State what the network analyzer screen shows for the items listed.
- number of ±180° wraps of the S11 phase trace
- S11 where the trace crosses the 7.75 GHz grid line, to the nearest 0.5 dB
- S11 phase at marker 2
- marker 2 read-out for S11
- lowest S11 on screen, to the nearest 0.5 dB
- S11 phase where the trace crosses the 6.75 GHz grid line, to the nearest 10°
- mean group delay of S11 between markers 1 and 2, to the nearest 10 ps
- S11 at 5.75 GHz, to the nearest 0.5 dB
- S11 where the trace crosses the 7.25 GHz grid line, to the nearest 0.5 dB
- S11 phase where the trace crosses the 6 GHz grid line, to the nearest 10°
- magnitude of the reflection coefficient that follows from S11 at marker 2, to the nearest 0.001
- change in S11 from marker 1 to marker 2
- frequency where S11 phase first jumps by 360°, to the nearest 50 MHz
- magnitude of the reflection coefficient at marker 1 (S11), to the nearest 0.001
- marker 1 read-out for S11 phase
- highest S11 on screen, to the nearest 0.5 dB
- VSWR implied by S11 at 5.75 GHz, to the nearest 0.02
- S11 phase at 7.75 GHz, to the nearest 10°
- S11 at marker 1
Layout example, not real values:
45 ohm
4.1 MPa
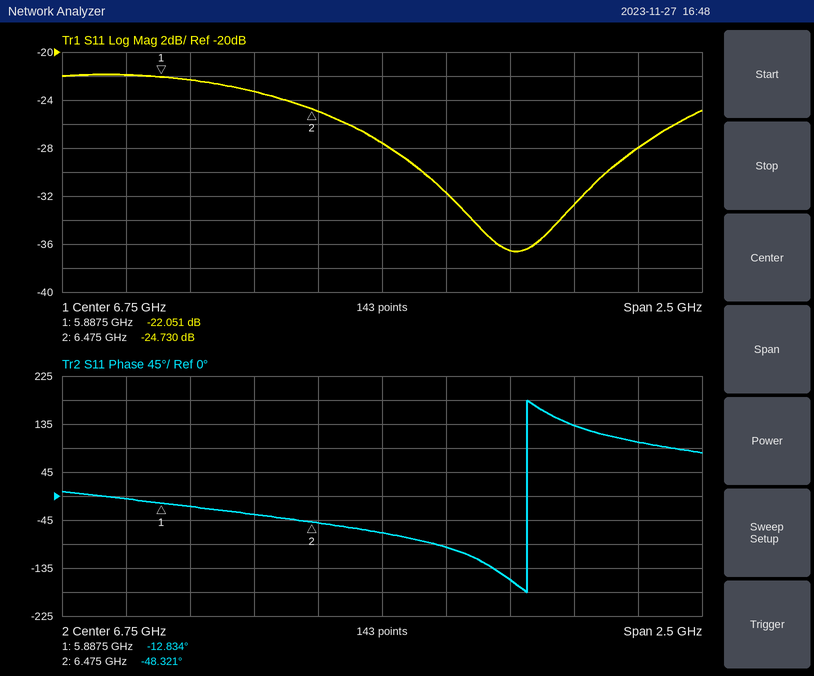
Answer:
1
-28.0 dB
-48.321°
-24.730 dB
-36.5 dB
-70°
170 ps
-22.0 dB
-36.5 dB
-20°
0.058
-2.679 dB
7.30 GHz
0.079
-12.834°
-22.0 dB
1.18
100°
-22.051 dB
